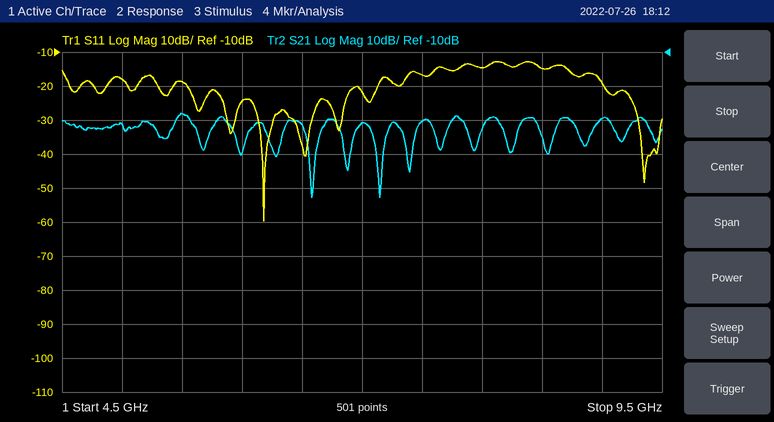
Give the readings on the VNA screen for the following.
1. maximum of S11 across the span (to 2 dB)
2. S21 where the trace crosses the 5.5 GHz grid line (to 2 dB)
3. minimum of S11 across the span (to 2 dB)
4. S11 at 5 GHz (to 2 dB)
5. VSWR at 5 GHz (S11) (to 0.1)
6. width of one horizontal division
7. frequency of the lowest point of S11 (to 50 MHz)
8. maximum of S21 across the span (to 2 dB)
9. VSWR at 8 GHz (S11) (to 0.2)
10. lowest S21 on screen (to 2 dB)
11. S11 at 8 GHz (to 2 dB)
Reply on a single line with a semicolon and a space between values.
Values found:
-12 dB; -28 dB; -60 dB; -18 dB; 1.3; 500 MHz; 6.20 GHz; -28 dB; 1.4; -52 dB; -14 dB
